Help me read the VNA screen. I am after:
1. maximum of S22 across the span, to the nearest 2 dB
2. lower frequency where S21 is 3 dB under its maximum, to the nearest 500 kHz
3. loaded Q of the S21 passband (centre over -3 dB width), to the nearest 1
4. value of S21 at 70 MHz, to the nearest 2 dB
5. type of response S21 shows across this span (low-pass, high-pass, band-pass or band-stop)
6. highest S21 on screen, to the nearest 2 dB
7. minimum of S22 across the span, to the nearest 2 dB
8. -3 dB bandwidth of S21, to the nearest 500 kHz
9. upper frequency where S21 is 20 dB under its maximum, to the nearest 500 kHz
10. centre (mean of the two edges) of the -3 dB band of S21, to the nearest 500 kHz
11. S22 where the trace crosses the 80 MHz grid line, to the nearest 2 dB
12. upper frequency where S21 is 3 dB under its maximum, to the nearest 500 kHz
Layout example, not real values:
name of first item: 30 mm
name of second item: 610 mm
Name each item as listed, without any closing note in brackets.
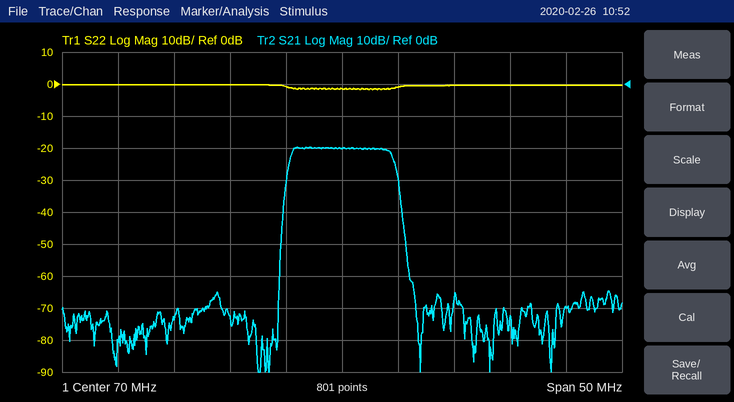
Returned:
maximum of S22 across the span, to the nearest 2 dB: 0 dB
lower frequency where S21 is 3 dB under its maximum, to the nearest 500 kHz: 65.5 MHz
loaded Q of the S21 passband (centre over -3 dB width), to the nearest 1: 8
value of S21 at 70 MHz, to the nearest 2 dB: -20 dB
type of response S21 shows across this span: band-pass
highest S21 on screen, to the nearest 2 dB: -20 dB
minimum of S22 across the span, to the nearest 2 dB: -2 dB
-3 dB bandwidth of S21, to the nearest 500 kHz: 9.0 MHz
upper frequency where S21 is 20 dB under its maximum, to the nearest 500 kHz: 75.5 MHz
centre (mean of the two edges) of the -3 dB band of S21, to the nearest 500 kHz: 70.0 MHz
S22 where the trace crosses the 80 MHz grid line, to the nearest 2 dB: 0 dB
upper frequency where S21 is 3 dB under its maximum, to the nearest 500 kHz: 74.5 MHz
